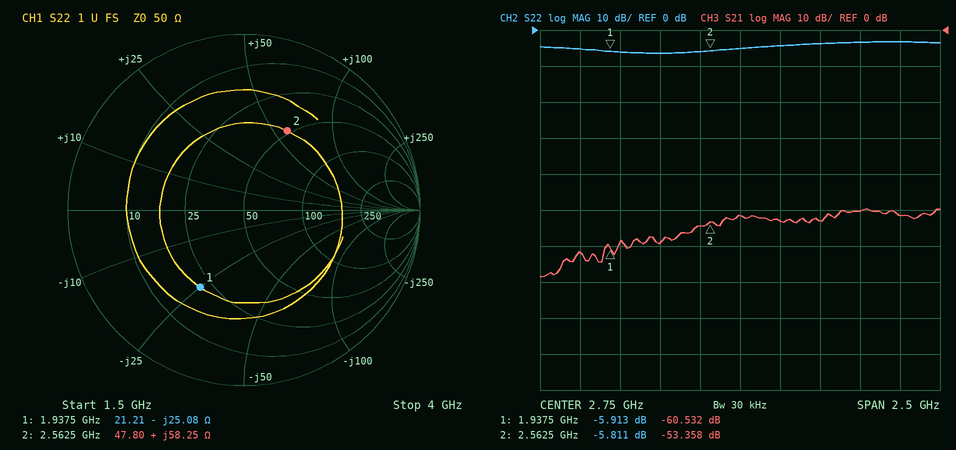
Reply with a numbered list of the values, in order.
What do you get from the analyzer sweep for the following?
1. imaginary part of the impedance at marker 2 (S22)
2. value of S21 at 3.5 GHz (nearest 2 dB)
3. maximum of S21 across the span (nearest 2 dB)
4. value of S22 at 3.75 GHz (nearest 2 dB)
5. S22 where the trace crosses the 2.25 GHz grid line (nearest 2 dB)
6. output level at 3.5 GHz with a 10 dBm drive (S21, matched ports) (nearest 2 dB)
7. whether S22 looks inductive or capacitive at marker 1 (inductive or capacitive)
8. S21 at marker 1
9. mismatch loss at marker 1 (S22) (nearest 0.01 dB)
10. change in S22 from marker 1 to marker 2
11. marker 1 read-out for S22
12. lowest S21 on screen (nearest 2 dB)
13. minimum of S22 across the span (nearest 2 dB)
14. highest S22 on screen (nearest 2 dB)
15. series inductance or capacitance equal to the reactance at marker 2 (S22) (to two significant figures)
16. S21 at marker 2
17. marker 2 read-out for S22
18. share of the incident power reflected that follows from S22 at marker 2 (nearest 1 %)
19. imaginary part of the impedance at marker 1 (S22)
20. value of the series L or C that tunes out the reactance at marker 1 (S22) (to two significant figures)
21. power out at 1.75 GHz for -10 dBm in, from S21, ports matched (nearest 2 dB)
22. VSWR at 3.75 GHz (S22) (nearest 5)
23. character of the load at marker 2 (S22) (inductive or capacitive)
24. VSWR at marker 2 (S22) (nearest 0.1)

1. +58.25 Ω
2. -50 dB
3. -50 dB
4. -4 dB
5. -6 dB
6. -40 dBm
7. capacitive
8. -60.532 dB
9. 1.29 dB
10. 0.102 dB
11. -5.913 dB
12. -68 dB
13. -6 dB
14. -4 dB
15. 3.6 nH
16. -53.358 dB
17. -5.811 dB
18. 26 %
19. -25.08 Ω
20. 2.1 nH
21. -72 dBm
22. 5
23. inductive
24. 3.1
